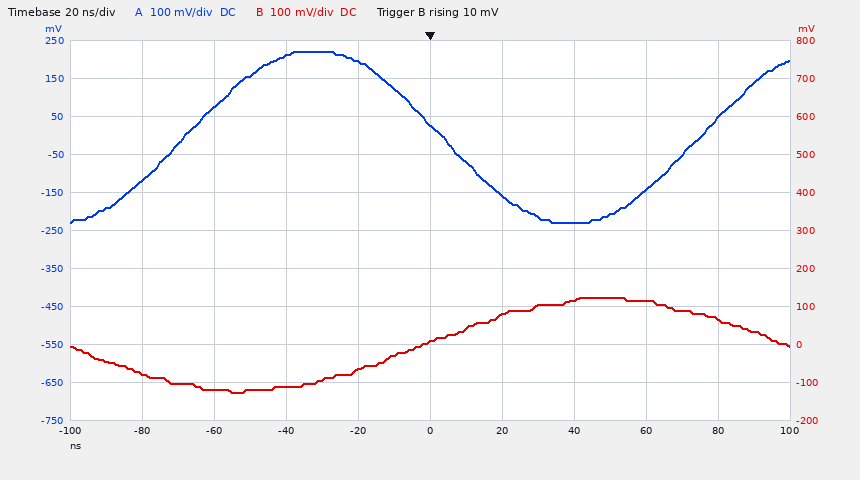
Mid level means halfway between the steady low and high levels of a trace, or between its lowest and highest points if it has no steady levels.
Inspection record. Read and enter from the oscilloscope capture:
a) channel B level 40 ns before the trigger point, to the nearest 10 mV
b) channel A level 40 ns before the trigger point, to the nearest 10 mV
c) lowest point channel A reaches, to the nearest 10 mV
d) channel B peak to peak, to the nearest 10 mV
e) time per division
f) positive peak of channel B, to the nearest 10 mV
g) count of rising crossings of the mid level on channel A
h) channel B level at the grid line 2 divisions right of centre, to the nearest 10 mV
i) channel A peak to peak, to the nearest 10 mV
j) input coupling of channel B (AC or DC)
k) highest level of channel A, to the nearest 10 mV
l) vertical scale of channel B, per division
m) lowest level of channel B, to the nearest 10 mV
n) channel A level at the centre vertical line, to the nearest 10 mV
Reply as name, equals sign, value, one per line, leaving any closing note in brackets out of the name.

channel B level 40 ns before the trigger point, to the nearest 10 mV = -110 mV
channel A level 40 ns before the trigger point, to the nearest 10 mV = 210 mV
lowest point channel A reaches, to the nearest 10 mV = -230 mV
channel B peak to peak, to the nearest 10 mV = 250 mV
time per division = 20 ns
positive peak of channel B, to the nearest 10 mV = 120 mV
count of rising crossings of the mid level on channel A = 2
channel B level at the grid line 2 divisions right of centre, to the nearest 10 mV = 120 mV
channel A peak to peak, to the nearest 10 mV = 450 mV
input coupling of channel B = DC
highest level of channel A, to the nearest 10 mV = 220 mV
vertical scale of channel B, per division = 100 mV
lowest level of channel B, to the nearest 10 mV = -130 mV
channel A level at the centre vertical line, to the nearest 10 mV = 30 mV
